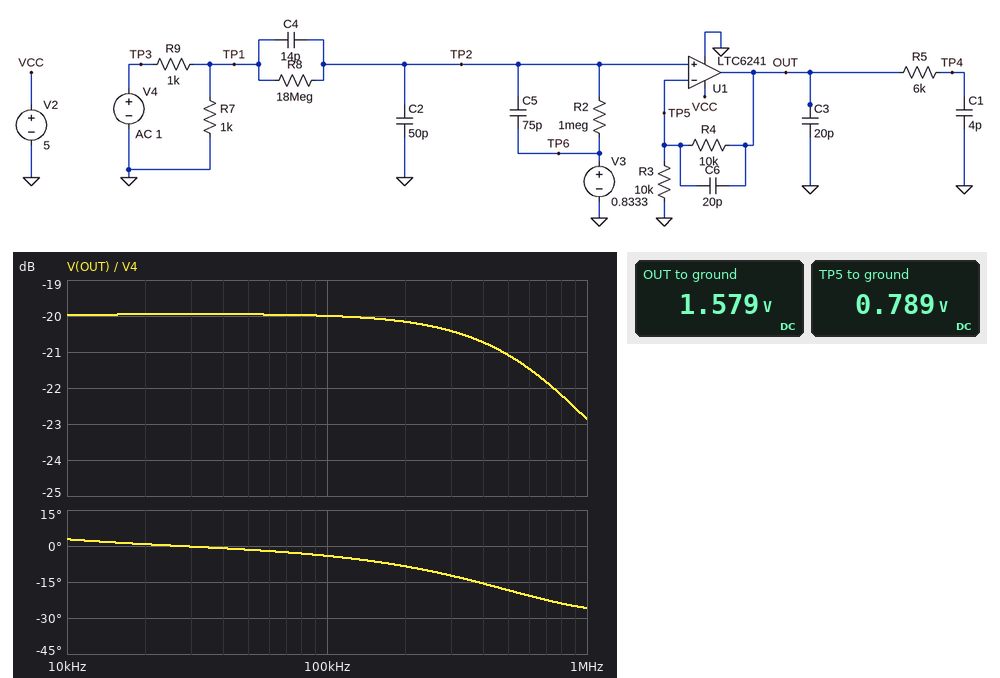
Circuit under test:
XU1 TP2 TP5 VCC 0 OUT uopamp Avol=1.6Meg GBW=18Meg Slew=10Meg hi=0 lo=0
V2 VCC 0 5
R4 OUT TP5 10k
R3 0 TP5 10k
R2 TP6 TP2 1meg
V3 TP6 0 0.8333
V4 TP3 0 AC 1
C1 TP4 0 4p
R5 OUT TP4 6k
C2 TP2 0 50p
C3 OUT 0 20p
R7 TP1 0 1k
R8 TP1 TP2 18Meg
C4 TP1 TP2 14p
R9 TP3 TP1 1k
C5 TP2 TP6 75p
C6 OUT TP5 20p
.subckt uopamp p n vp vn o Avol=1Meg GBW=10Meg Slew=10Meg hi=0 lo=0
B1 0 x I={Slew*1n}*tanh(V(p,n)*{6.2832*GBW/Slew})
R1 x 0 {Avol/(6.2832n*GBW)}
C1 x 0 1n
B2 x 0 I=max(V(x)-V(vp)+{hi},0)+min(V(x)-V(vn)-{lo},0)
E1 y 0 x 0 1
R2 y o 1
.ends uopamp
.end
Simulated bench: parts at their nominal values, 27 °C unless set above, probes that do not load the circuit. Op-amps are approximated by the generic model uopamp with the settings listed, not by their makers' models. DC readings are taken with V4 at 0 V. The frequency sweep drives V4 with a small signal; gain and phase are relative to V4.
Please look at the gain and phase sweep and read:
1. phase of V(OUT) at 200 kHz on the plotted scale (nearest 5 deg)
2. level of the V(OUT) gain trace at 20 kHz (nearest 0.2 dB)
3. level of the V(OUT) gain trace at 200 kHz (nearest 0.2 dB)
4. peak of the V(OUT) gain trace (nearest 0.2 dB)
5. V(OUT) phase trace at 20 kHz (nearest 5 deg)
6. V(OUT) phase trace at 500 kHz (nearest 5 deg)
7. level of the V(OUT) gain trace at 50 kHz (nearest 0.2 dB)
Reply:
-10 deg
-20.0 dB
-20.2 dB
-20.0 dB
0 deg
-20 deg
-20.0 dB
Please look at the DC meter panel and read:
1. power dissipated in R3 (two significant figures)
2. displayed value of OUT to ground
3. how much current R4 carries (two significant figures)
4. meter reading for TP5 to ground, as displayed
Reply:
62 µW
1.579 V
79 µA
0.789 V
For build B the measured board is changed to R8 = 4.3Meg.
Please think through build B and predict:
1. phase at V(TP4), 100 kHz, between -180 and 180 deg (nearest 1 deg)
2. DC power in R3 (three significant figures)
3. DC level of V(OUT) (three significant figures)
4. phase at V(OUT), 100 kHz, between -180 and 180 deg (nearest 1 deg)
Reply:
-6 deg
45.7 µW
1.35 V
-5 deg
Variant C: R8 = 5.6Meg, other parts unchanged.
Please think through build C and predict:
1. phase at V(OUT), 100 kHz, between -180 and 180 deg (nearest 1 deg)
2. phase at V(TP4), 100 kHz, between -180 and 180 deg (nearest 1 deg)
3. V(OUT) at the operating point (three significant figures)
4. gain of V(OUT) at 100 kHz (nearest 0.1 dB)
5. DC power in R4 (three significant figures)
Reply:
-5 deg
-6 deg
1.41 V
-20.0 dB
50.0 µW
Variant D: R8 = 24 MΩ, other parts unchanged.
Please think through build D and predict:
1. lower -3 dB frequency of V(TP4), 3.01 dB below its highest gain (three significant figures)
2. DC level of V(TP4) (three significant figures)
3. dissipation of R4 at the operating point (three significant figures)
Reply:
984 Hz
1.60 V
64.0 µW
